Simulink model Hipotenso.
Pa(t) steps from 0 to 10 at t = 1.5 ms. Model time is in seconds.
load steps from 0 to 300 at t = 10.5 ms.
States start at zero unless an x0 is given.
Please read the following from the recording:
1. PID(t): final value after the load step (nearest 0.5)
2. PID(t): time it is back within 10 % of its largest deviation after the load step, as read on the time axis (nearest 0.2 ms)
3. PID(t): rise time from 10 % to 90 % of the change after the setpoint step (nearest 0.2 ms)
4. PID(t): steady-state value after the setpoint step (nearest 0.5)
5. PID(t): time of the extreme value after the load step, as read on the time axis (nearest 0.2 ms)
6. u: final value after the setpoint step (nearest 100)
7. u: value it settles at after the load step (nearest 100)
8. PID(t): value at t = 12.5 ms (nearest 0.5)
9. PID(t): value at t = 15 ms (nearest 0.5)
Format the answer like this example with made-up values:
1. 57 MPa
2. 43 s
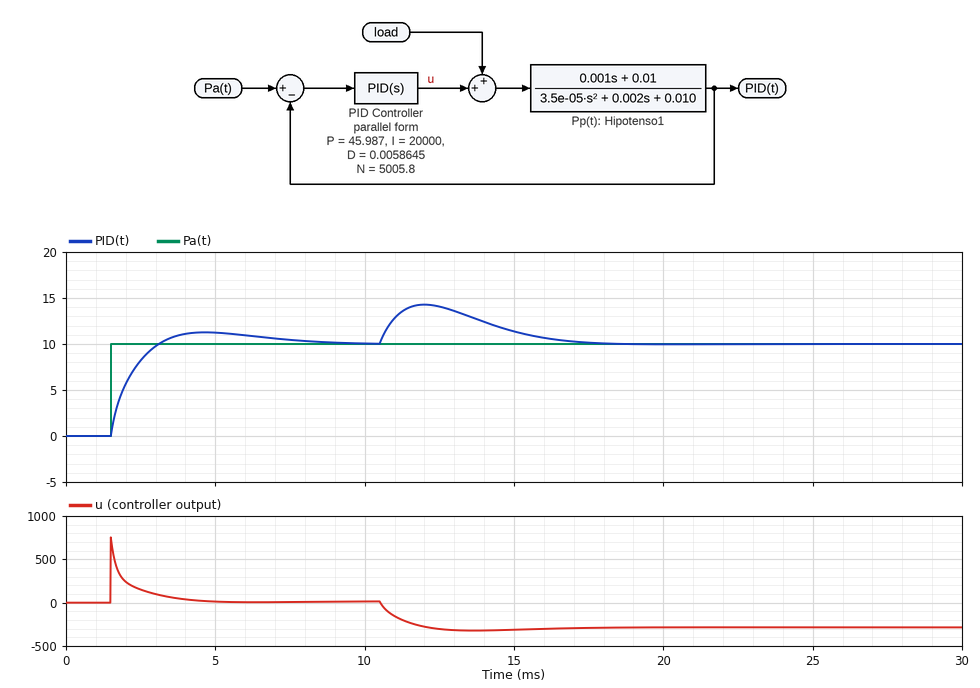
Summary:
1. 10.0
2. 16.6 ms
3. 1.2 ms
4. 10.0
5. 12.0 ms
6. 0
7. -300
8. 14.0
9. 11.5
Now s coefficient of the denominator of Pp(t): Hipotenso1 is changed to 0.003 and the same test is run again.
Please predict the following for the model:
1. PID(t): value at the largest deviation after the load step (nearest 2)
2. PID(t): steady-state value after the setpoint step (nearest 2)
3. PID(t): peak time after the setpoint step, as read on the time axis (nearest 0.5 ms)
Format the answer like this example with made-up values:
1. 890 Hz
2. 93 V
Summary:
1. 14
2. 10
3. 4.5 ms
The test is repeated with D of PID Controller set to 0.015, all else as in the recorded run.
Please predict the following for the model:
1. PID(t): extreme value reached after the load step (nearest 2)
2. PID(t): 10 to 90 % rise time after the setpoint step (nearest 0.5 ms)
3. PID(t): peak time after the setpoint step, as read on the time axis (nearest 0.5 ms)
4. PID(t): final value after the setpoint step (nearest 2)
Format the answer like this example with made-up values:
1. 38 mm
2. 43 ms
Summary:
1. 14
2. 1.5 ms
3. 5.0 ms
4. 10
